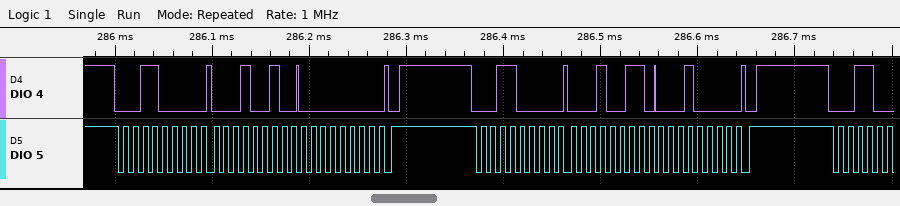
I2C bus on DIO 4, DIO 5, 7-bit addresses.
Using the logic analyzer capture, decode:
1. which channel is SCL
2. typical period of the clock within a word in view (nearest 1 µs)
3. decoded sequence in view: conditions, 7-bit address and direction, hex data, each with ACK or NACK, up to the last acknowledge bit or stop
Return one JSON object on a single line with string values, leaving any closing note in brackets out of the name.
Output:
{"which channel is SCL": "DIO 5", "typical period of the clock within a word in view": "10 µs", "decoded sequence in view: conditions, 7-bit address and direction, hex data, each with ACK or NACK, up to the last acknowledge bit or stop": "start, address 18 write ACK, 12 ACK, 00 ACK, stop, start, address 18 write ACK, 13 ACK, 10 ACK, stop"}
